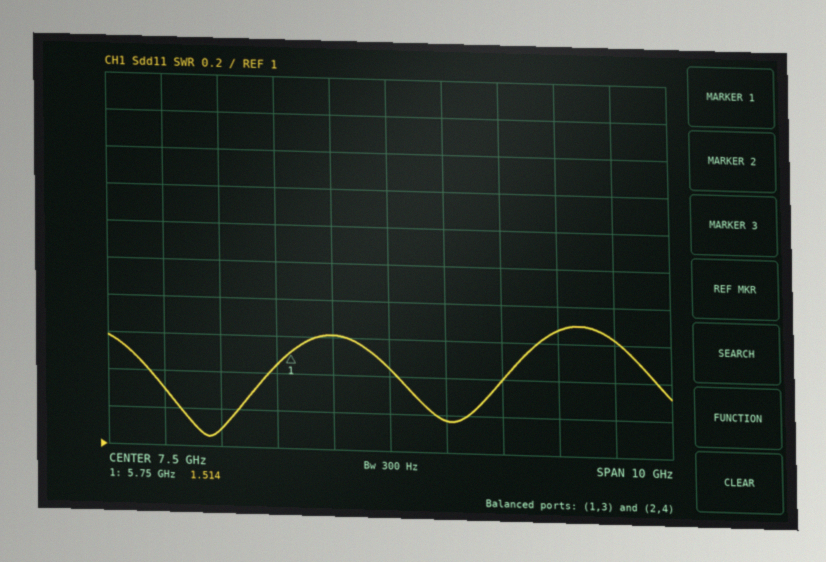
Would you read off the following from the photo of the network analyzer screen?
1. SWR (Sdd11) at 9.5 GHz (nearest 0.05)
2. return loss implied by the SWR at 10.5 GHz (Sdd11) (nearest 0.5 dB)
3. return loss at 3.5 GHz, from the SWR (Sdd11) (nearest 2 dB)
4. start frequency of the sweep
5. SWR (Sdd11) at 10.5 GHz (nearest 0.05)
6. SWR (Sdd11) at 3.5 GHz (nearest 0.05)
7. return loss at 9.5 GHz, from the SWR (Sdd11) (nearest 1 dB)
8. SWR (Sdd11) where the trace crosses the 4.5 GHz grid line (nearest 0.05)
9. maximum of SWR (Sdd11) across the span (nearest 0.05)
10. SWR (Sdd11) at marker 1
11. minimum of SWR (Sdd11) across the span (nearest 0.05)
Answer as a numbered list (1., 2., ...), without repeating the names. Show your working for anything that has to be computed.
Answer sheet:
1. 1.40
2. −20 log10((1.65 − 1)/(1.65 + 1)) ≈ 12.2 dB, so 12.0 dB to the nearest 0.5 dB
3. −20 log10((1.3 − 1)/(1.3 + 1)) ≈ 18 dB
4. 2.5 GHz
5. 1.65
6. 1.30
7. −20 log10((1.4 − 1)/(1.4 + 1)) ≈ 16 dB
8. 1.10
9. 1.70
10. 1.514
11. 1.05
